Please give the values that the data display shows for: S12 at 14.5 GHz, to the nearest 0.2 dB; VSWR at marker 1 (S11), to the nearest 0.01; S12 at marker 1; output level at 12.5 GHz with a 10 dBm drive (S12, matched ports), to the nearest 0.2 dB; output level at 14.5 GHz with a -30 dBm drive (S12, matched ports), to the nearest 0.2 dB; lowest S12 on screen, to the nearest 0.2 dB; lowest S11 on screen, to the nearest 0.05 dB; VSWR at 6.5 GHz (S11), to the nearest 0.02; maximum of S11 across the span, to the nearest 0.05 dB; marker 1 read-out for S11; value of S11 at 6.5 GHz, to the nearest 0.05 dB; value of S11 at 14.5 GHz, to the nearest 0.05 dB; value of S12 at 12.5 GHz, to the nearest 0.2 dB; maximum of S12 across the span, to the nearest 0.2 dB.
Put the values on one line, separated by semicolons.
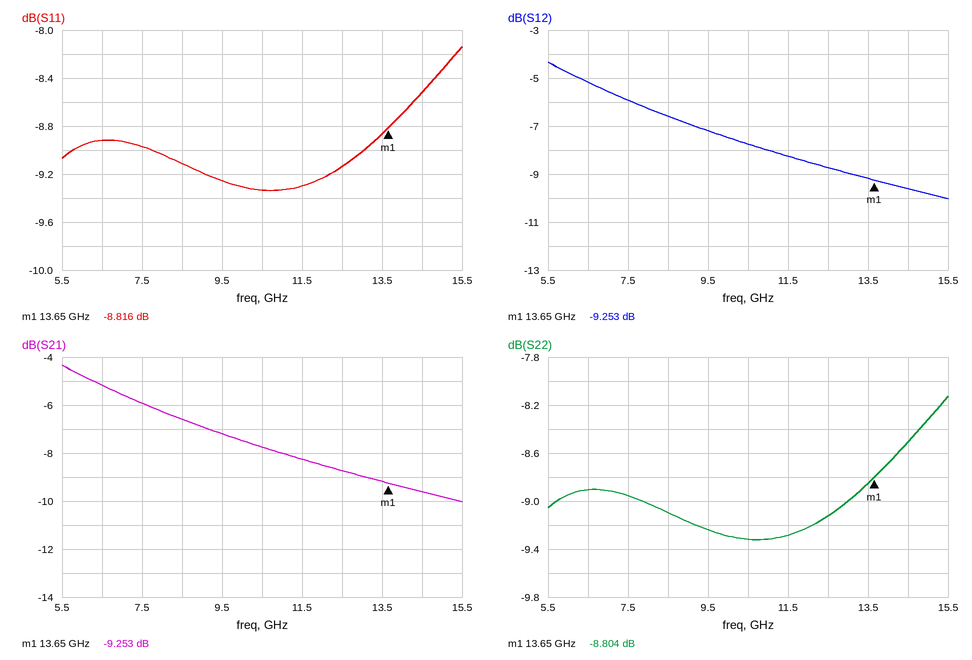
-9.6 dB; 2.14; -9.253 dB; 1.2 dBm; -39.6 dBm; -10.0 dB; -9.35 dB; 2.12; -8.15 dB; -8.816 dB; -8.90 dB; -8.50 dB; -8.8 dB; -4.4 dB
